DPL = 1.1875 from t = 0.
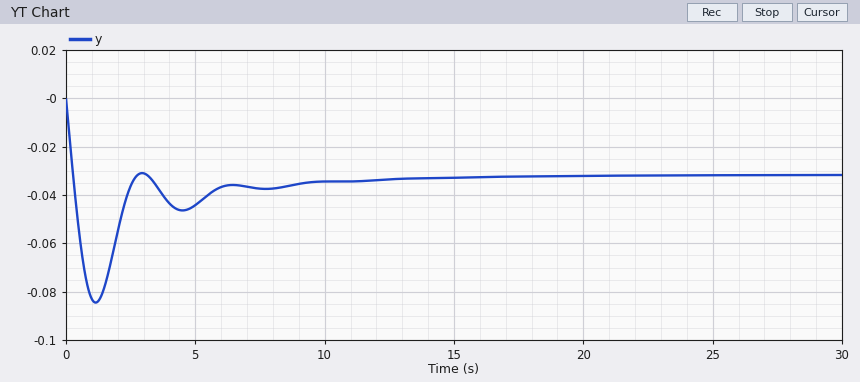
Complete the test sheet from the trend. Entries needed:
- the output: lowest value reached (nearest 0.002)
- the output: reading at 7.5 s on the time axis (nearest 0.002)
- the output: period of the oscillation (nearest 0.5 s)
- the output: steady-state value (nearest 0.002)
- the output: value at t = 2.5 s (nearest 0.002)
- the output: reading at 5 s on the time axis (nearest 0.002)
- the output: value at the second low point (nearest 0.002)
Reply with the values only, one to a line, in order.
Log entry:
-0.084
-0.038
3.5 s
-0.032
-0.036
-0.044
-0.046
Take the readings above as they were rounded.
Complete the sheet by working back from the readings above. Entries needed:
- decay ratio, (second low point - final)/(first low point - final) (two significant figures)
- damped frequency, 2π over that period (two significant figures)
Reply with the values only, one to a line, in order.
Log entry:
0.27
1.8 rad/s
